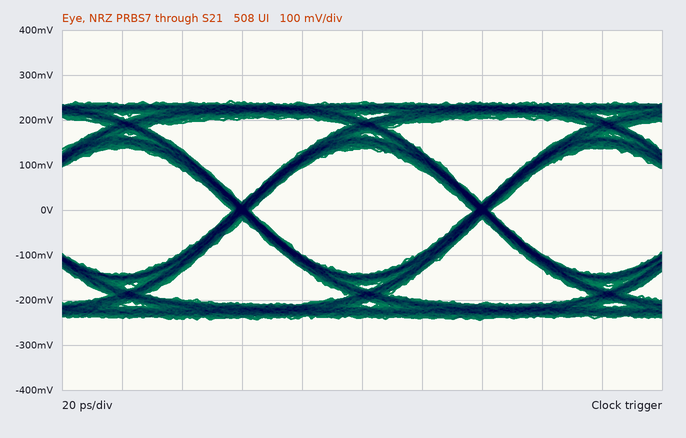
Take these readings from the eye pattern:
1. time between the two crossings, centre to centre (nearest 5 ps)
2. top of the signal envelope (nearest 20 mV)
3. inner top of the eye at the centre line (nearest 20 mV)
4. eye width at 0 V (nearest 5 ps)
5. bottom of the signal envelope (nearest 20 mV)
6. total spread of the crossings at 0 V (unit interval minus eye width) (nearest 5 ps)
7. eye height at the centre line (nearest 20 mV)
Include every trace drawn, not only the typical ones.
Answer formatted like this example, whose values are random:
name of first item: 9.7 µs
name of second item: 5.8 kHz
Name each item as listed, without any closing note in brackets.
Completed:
time between the two crossings, centre to centre: 80 ps
top of the signal envelope: 240 mV
inner top of the eye at the centre line: 140 mV
eye width at 0 V: 75 ps
bottom of the signal envelope: -240 mV
total spread of the crossings at 0 V (unit interval minus eye width): 5 ps
eye height at the centre line: 280 mV
